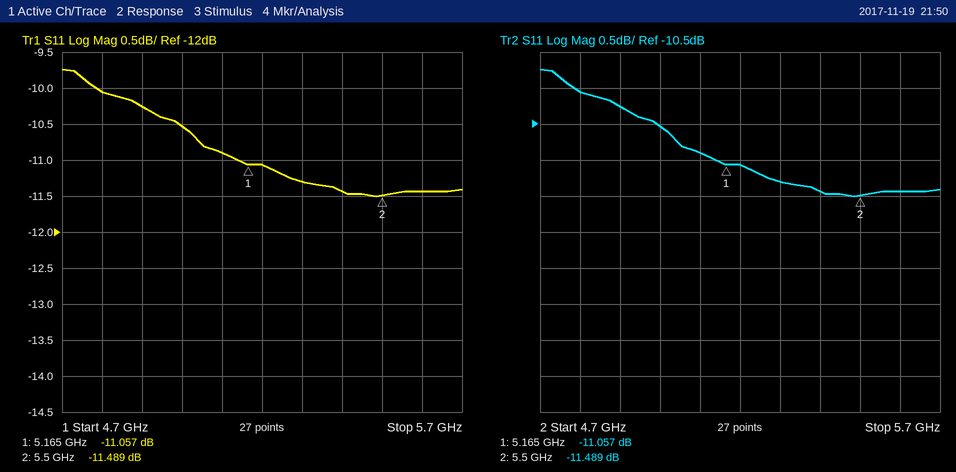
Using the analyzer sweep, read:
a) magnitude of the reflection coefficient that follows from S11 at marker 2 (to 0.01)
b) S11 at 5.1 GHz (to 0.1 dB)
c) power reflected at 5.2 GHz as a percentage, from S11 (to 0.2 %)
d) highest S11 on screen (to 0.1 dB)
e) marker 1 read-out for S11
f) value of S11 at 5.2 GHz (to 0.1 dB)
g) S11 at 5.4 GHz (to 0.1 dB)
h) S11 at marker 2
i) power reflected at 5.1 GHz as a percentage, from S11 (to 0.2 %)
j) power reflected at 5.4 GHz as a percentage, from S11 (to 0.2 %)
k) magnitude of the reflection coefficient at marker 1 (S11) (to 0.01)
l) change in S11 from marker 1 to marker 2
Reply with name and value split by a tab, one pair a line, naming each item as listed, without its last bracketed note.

magnitude of the reflection coefficient that follows from S11 at marker 2	0.27
S11 at 5.1 GHz	-10.9 dB
power reflected at 5.2 GHz as a percentage, from S11	7.8 %
highest S11 on screen	-9.7 dB
marker 1 read-out for S11	-11.057 dB
value of S11 at 5.2 GHz	-11.1 dB
S11 at 5.4 GHz	-11.4 dB
S11 at marker 2	-11.489 dB
power reflected at 5.1 GHz as a percentage, from S11	8.2 %
power reflected at 5.4 GHz as a percentage, from S11	7.2 %
magnitude of the reflection coefficient at marker 1 (S11)	0.28
change in S11 from marker 1 to marker 2	-0.432 dB
